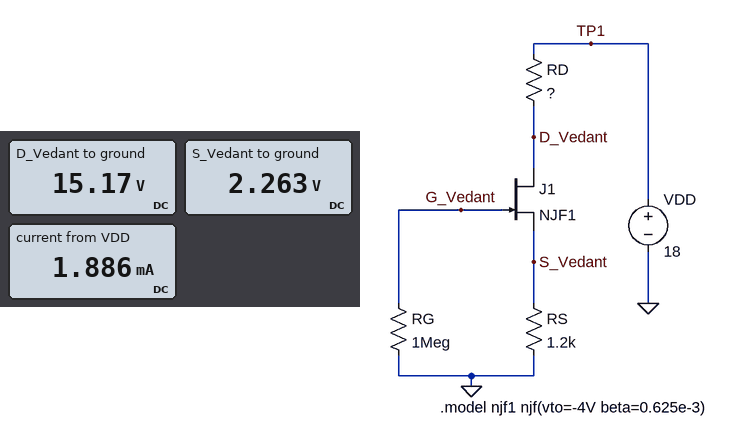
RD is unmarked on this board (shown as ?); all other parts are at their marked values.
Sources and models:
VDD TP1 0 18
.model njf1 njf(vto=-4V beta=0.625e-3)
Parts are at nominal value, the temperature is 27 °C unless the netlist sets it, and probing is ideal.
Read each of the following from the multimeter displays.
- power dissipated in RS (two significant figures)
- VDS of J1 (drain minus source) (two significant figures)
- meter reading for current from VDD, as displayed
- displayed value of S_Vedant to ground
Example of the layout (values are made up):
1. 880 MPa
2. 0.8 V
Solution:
1. 4.3 mW
2. 13 V
3. 1.886 mA
4. 2.263 V
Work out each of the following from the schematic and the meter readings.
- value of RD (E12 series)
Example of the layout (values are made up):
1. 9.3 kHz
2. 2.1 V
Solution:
1. 1.5 kΩ
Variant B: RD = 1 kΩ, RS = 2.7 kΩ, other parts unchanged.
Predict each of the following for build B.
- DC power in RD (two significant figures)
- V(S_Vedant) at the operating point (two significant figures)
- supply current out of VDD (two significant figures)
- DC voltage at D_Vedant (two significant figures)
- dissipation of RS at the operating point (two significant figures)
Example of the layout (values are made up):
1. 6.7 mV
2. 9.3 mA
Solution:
1. 1.0 mW
2. 2.7 V
3. 1.0 mA
4. 17 V
5. 2.8 mW
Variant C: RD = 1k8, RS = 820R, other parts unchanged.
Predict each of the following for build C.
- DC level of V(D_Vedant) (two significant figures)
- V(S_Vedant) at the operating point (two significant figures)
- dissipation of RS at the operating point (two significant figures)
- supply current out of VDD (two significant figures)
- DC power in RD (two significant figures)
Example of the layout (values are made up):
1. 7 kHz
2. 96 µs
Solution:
1. 14 V
2. 2.0 V
3. 5.0 mW
4. 2.5 mA
5. 11 mW
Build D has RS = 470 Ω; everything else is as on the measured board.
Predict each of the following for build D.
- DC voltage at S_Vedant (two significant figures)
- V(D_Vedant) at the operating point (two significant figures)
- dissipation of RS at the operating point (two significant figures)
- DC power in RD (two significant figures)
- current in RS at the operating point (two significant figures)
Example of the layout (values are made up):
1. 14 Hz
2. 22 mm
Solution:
1. 1.6 V
2. 13 V
3. 5.7 mW
4. 18 mW
5. 3.5 mA
